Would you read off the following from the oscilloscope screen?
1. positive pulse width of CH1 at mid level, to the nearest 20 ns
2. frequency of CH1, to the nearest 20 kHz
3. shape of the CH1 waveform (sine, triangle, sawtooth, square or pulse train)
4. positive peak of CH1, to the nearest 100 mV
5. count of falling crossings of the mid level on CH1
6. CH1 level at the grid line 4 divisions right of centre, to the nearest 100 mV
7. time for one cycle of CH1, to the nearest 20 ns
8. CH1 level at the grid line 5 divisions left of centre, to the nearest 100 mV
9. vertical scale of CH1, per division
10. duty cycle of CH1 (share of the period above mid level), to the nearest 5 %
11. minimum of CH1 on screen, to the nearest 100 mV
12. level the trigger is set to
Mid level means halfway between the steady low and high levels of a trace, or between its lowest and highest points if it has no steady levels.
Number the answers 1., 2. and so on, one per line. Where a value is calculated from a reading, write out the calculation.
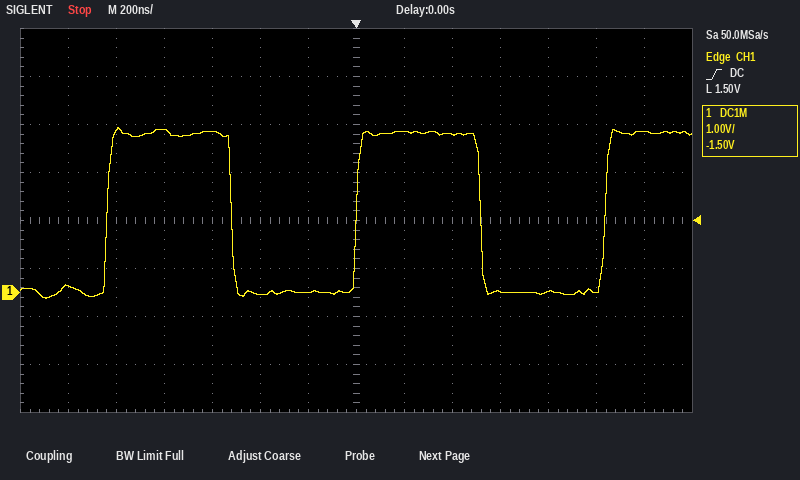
1. 520 ns
2. 1 / 1.04 µs ≈ 962 kHz, so 960 kHz to the nearest 20 kHz
3. square
4. 3.4 V
5. 2
6. 0.0 V
7. 1.04 µs
8. 3.4 V
9. 1 V
10. 520 ns / 1.04 µs ≈ 50 %
11. -100 mV
12. 1.50 V
